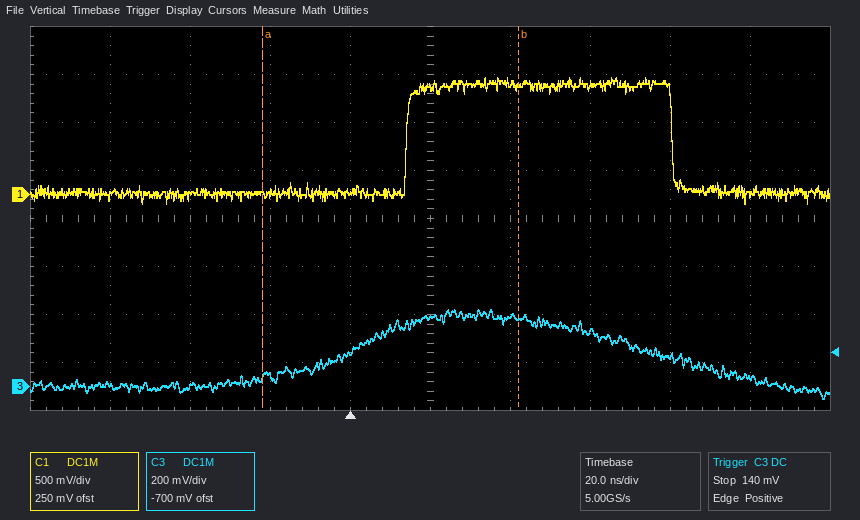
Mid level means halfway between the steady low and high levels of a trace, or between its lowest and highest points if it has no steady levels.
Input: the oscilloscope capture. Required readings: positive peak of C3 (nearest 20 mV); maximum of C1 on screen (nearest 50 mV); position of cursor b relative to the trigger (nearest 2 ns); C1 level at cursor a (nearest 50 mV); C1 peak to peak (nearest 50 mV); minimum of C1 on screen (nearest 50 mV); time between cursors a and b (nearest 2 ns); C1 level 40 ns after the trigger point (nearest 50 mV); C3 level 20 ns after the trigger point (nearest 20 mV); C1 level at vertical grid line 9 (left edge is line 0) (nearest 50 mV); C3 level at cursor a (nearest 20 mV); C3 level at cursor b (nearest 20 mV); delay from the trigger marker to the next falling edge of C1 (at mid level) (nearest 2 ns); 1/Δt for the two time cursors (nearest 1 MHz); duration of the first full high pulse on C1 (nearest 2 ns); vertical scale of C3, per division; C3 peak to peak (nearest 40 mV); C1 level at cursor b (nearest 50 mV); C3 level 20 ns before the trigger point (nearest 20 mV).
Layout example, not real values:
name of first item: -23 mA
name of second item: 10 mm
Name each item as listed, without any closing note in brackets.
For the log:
positive peak of C3: 320 mV
maximum of C1 on screen: 1.20 V
position of cursor b relative to the trigger: +42 ns
C1 level at cursor a: 0 mV
C1 peak to peak: 1.30 V
minimum of C1 on screen: -100 mV
time between cursors a and b: 64 ns
C1 level 40 ns after the trigger point: 1.15 V
C3 level 20 ns after the trigger point: 280 mV
C1 level at vertical grid line 9 (left edge is line 0): 0 mV
C3 level at cursor a: 40 mV
C3 level at cursor b: 280 mV
delay from the trigger marker to the next falling edge of C1 (at mid level): 80 ns
1/Δt for the two time cursors: 16 MHz
duration of the first full high pulse on C1: 66 ns
vertical scale of C3, per division: 200 mV
C3 peak to peak: 360 mV
C1 level at cursor b: 1.10 V
C3 level 20 ns before the trigger point: 40 mV
